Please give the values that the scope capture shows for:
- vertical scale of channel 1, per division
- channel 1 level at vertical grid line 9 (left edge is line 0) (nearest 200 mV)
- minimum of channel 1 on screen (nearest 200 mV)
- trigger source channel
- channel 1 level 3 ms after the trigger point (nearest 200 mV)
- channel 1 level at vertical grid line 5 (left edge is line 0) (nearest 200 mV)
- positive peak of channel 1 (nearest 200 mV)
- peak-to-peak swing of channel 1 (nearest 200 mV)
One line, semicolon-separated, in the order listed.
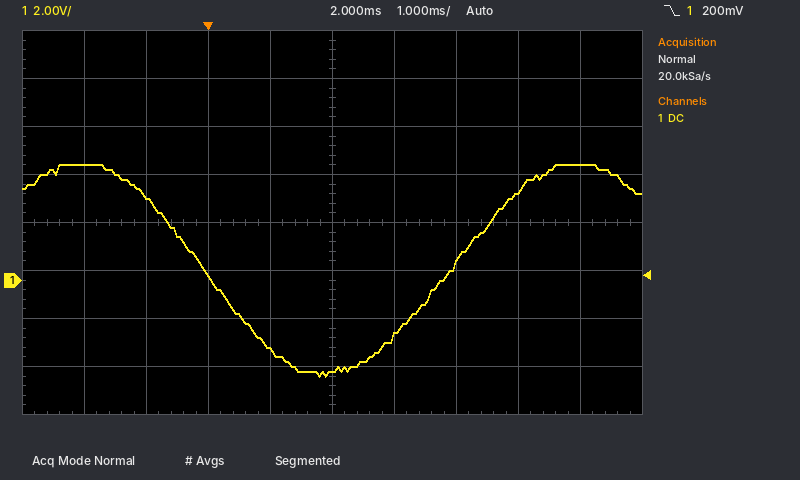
2 V; 4.8 V; -4.0 V; channel 1; -2.4 V; -3.8 V; 4.8 V; 8.8 V
